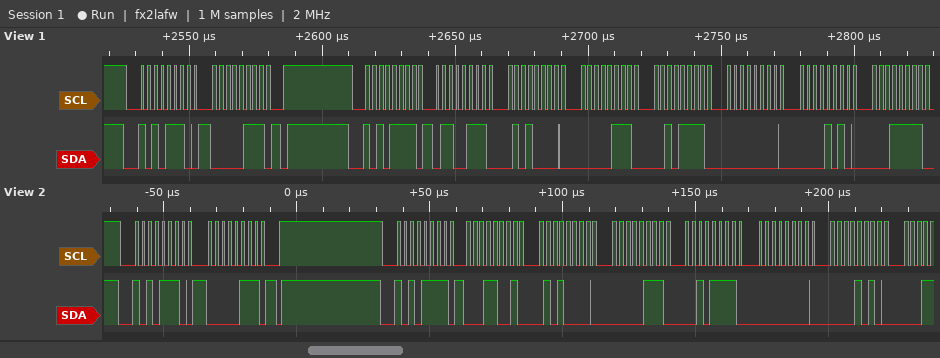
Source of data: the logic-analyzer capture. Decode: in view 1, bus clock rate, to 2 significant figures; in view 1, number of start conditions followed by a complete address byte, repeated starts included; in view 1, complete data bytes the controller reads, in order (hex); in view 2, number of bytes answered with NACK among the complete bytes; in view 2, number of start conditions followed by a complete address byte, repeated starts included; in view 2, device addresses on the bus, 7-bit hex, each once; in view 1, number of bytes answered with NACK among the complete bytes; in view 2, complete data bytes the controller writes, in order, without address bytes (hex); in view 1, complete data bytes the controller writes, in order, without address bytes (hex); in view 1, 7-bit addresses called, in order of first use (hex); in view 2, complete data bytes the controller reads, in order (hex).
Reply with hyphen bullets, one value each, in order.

- 400 kHz
- 2
- 67 50 07 2F 00 0A 1F
- 0
- 2
- 0x57
- 0
- 07
- 07
- 0x57
- 19 50 07 2F 00 0A
